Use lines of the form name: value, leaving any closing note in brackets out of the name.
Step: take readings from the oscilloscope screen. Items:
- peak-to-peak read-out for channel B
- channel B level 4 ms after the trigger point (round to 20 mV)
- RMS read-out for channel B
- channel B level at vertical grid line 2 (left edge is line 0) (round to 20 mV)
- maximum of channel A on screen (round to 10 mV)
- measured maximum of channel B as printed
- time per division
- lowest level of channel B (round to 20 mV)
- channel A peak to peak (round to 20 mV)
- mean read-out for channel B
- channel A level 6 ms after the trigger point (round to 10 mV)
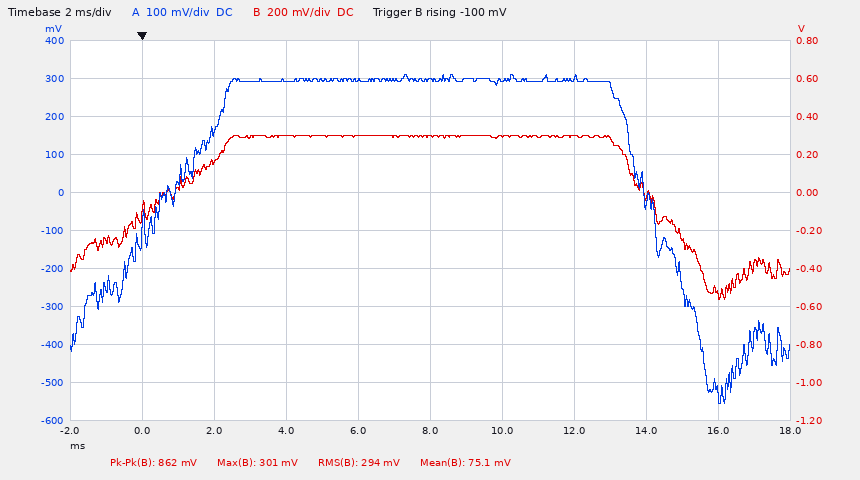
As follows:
peak-to-peak read-out for channel B: 862 mV
channel B level 4 ms after the trigger point: 300 mV
RMS read-out for channel B: 294 mV
channel B level at vertical grid line 2 (left edge is line 0): 160 mV
maximum of channel A on screen: 310 mV
measured maximum of channel B as printed: 301 mV
time per division: 2 ms
lowest level of channel B: -560 mV
channel A peak to peak: 860 mV
mean read-out for channel B: 75.1 mV
channel A level 6 ms after the trigger point: 300 mV
